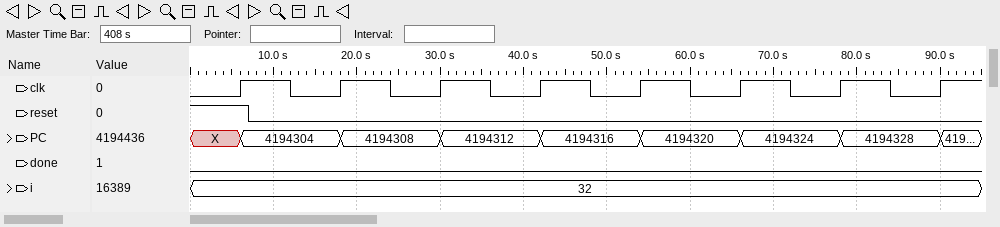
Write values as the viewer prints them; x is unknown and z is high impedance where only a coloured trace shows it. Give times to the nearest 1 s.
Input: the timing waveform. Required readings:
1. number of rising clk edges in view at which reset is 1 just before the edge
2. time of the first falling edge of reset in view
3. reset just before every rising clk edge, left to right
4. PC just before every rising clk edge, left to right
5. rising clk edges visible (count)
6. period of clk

1
7 s
1 0 0 0 0 0 0 0
X, 4194304, 4194308, 4194312, 4194316, 4194320, 4194324, 4194328
8
12 s
